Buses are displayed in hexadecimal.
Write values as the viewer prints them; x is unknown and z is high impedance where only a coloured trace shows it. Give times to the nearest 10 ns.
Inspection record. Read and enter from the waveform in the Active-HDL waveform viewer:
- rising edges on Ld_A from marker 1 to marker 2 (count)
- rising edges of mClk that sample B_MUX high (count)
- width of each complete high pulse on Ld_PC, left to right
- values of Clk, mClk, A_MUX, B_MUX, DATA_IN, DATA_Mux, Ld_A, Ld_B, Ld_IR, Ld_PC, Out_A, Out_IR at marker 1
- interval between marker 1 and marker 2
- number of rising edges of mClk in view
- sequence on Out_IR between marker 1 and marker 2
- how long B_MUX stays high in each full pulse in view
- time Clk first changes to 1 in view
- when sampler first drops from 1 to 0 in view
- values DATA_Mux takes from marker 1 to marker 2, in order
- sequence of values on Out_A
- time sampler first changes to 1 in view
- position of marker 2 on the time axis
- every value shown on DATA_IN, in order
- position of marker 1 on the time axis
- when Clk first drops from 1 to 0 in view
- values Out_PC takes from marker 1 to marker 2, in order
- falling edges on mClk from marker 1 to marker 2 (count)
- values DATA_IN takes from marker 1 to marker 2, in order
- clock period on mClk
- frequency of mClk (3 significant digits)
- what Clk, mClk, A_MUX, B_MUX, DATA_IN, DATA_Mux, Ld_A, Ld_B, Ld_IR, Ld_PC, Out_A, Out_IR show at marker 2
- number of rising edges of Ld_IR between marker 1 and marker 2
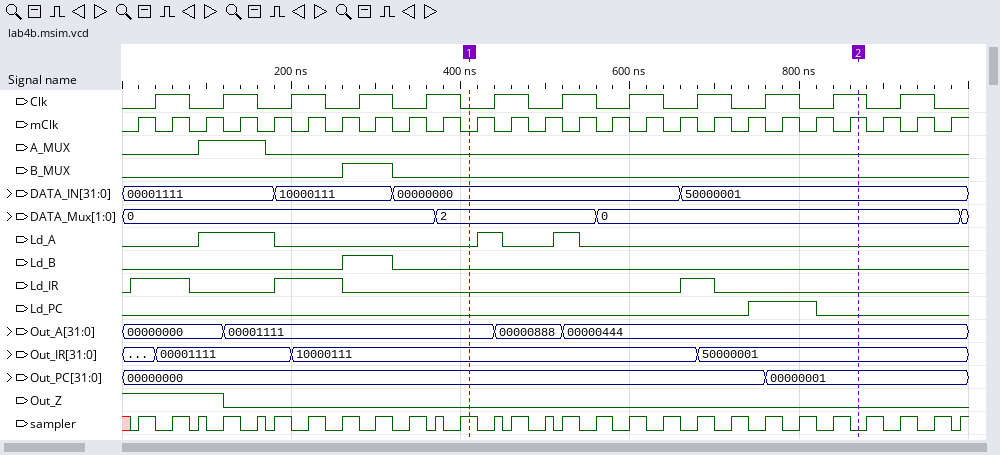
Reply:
2
1
80 ns
Clk=0, mClk=0, A_MUX=0, B_MUX=0, DATA_IN=00000000, DATA_Mux=2, Ld_A=0, Ld_B=0, Ld_IR=0, Ld_PC=0, Out_A=00001111, Out_IR=10000111
460 ns
25
10000111, 50000001
60 ns
40 ns
40 ns
2, 0
00000000, 00001111, 00000888, 00000444
20 ns
870 ns
00001111, 10000111, 00000000, 50000001
410 ns
80 ns
00000000, 00000001
11
00000000, 50000001
40 ns
25.0 MHz
Clk=1, mClk=1, A_MUX=0, B_MUX=0, DATA_IN=50000001, DATA_Mux=0, Ld_A=0, Ld_B=0, Ld_IR=0, Ld_PC=0, Out_A=00000444, Out_IR=50000001
1
